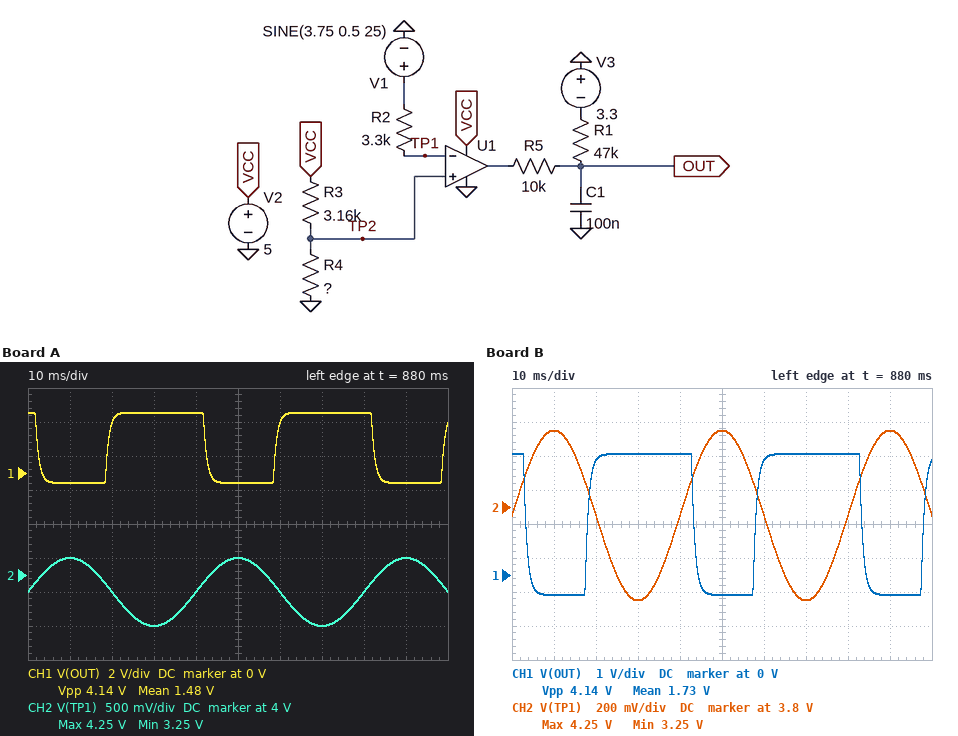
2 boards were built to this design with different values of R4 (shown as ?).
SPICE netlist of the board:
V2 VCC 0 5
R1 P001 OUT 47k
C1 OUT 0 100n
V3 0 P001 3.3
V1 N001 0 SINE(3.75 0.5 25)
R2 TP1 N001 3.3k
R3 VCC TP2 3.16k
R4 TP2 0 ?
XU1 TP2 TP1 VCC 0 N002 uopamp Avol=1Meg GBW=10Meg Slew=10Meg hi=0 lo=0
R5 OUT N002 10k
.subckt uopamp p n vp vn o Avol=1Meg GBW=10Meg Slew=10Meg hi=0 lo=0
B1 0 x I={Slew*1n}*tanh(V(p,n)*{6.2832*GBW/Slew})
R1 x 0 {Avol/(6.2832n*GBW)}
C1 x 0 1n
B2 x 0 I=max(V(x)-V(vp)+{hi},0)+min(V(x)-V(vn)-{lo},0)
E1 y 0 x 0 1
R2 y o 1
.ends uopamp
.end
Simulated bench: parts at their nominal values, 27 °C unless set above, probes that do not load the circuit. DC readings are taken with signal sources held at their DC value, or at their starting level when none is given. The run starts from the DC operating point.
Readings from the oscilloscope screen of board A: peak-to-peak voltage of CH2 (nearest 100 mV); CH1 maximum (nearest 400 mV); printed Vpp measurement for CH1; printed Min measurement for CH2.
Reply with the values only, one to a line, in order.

1.0 V
3.6 V
4.14 V
3.25 V
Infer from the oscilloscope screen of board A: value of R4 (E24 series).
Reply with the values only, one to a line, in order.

11 kΩ
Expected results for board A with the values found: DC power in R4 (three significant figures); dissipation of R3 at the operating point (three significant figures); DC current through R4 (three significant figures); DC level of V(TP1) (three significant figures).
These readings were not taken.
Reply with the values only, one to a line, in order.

1.37 mW
394 µW
353 µA
3.75 V
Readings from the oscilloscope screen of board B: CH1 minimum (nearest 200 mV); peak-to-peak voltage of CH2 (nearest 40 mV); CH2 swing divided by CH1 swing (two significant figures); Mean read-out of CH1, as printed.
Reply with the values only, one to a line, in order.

-600 mV
1.00 V
0.24
1.73 V
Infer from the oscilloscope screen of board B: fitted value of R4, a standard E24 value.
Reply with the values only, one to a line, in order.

12 kΩ
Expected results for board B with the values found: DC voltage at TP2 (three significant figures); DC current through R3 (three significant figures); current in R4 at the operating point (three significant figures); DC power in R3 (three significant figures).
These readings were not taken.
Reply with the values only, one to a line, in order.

3.96 V
330 µA
330 µA
344 µW
